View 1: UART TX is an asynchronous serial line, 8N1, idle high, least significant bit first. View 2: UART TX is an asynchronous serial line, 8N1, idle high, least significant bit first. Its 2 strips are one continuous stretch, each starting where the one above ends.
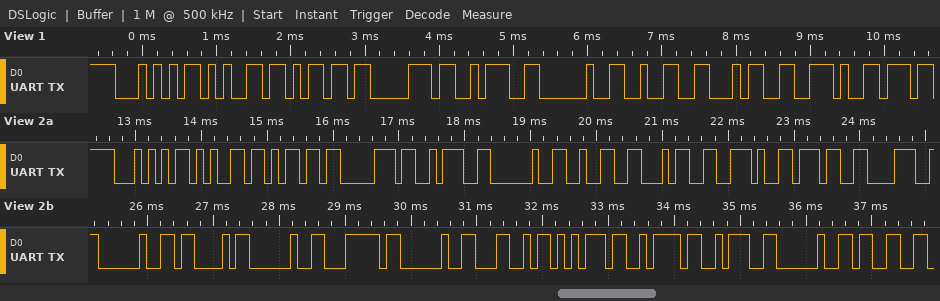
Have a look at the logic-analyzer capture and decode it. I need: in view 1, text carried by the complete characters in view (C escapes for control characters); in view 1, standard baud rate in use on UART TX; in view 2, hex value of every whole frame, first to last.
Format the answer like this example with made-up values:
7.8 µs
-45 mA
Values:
"Temp: 24."
9600 baud
54 65 6D 70 3A 20 32 34 2E 37 38 20 43 20 7C 20 4C 75 7A 3A 20 33
